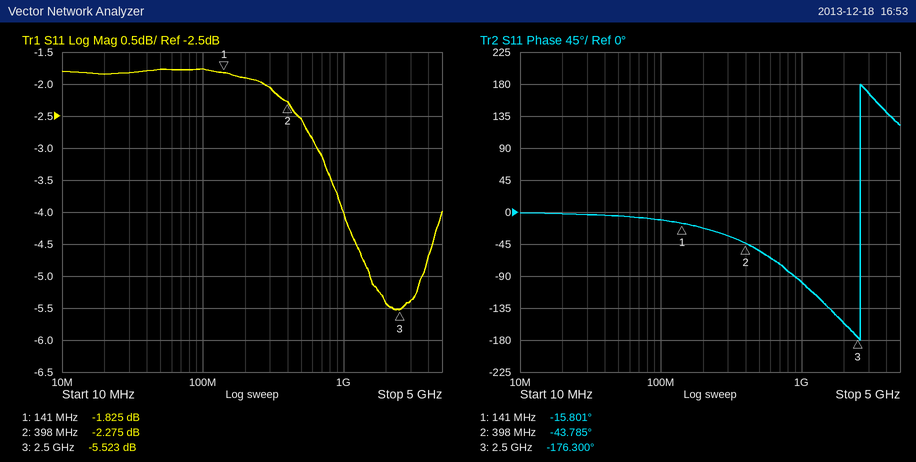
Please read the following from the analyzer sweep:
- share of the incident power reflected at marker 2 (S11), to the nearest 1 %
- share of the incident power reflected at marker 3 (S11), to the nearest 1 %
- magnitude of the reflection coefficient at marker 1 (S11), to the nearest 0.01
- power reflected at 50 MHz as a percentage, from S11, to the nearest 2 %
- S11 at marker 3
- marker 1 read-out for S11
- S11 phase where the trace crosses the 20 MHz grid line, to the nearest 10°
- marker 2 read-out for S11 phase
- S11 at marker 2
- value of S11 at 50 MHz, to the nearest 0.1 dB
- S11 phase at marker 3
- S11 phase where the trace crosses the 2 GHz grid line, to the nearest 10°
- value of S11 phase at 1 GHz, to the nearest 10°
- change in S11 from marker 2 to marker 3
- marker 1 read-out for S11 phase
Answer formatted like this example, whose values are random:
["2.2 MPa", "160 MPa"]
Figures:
["59 %", "28 %", "0.81", "66 %", "-5.523 dB", "-1.825 dB", "0°", "-43.785°", "-2.275 dB", "-1.8 dB", "-176.300°", "-160°", "-100°", "-3.248 dB", "-15.801°"]
